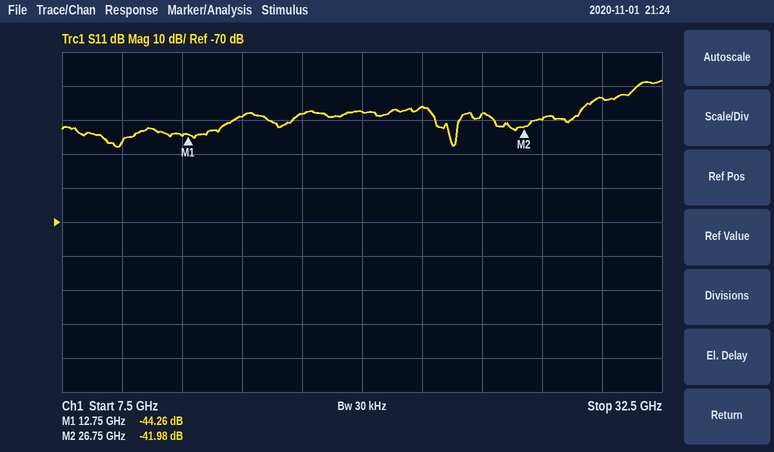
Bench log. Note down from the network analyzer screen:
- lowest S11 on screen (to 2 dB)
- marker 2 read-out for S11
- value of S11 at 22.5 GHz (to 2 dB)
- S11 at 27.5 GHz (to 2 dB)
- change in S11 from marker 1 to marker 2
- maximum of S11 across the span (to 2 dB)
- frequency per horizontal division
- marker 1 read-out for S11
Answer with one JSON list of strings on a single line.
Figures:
["-48 dB", "-41.98 dB", "-36 dB", "-40 dB", "2.28 dB", "-28 dB", "2.5 GHz", "-44.26 dB"]
